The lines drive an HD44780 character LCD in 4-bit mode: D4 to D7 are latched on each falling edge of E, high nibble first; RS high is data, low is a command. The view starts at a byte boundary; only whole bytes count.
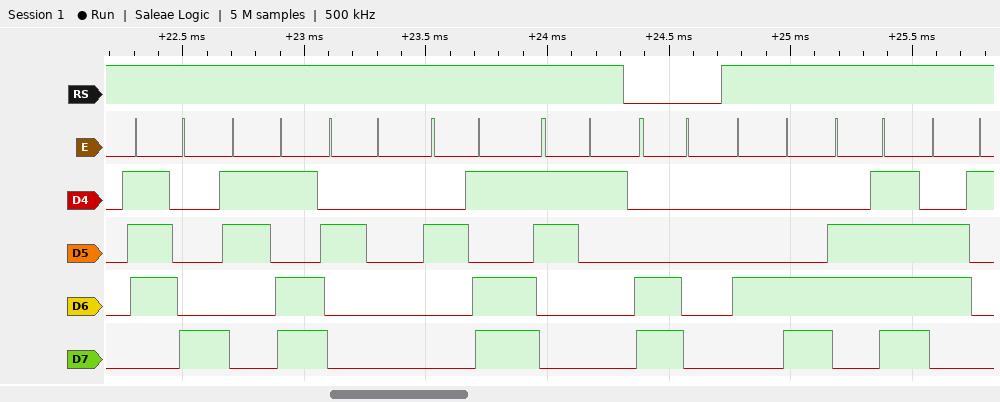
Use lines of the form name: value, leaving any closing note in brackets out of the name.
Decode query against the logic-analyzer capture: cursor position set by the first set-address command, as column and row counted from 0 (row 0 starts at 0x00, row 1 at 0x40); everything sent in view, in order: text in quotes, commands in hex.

cursor position set by the first set-address command, as column and row counted from 0: column 0, row 1
everything sent in view, in order: text in quotes, commands in hex: "x= -1" 0xC0 "Loa"
